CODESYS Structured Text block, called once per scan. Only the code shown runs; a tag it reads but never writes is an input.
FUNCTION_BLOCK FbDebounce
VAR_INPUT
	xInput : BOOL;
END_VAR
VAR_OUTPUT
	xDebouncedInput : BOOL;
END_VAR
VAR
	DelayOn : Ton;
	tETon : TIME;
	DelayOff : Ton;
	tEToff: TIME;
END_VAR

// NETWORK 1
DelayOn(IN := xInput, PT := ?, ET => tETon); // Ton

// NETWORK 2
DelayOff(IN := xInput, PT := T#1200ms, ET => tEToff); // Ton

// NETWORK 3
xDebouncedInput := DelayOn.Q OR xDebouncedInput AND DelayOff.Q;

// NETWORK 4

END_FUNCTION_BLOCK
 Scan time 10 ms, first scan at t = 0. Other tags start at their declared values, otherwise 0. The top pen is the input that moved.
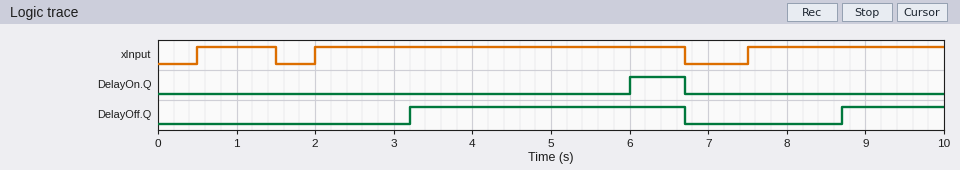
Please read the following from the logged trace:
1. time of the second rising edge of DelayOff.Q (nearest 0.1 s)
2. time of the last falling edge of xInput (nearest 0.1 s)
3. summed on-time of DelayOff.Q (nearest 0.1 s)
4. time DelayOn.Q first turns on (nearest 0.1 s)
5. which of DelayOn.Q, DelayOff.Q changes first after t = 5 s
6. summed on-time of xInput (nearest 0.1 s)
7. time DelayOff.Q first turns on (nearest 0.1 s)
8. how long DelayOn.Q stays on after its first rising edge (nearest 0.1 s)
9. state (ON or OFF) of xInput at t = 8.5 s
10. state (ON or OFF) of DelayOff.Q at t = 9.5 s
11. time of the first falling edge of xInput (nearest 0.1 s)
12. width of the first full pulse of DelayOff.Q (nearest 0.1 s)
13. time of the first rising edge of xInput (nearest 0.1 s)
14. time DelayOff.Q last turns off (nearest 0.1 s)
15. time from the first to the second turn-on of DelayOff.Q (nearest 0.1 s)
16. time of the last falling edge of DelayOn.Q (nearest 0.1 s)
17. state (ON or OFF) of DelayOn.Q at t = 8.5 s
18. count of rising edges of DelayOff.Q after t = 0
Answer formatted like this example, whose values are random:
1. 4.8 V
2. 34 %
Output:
1. 8.7 s
2. 6.7 s
3. 4.8 s
4. 6.0 s
5. DelayOn.Q
6. 8.2 s
7. 3.2 s
8. 0.7 s
9. ON
10. ON
11. 1.5 s
12. 3.5 s
13. 0.5 s
14. 6.7 s
15. 5.5 s
16. 6.7 s
17. OFF
18. 2
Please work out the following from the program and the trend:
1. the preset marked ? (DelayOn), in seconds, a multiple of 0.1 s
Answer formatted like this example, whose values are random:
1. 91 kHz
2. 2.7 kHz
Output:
1. 4.0 s
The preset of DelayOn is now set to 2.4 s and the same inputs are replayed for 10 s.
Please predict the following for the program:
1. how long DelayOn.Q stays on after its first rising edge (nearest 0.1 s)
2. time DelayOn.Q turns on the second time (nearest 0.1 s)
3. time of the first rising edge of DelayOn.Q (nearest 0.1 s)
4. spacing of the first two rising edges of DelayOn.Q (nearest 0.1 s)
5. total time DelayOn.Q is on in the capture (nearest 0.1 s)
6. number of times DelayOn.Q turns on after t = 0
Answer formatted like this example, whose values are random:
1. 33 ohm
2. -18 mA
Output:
1. 2.3 s
2. 9.9 s
3. 4.4 s
4. 5.5 s
5. 2.4 s
6. 2
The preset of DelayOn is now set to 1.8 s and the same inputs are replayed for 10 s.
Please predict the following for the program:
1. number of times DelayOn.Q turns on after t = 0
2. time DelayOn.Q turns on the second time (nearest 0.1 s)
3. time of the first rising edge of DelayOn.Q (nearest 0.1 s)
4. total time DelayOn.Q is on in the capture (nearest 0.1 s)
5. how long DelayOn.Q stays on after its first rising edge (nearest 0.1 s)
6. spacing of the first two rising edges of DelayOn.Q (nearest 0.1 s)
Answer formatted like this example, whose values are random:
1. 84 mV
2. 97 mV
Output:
1. 2
2. 9.3 s
3. 3.8 s
4. 3.6 s
5. 2.9 s
6. 5.5 s
